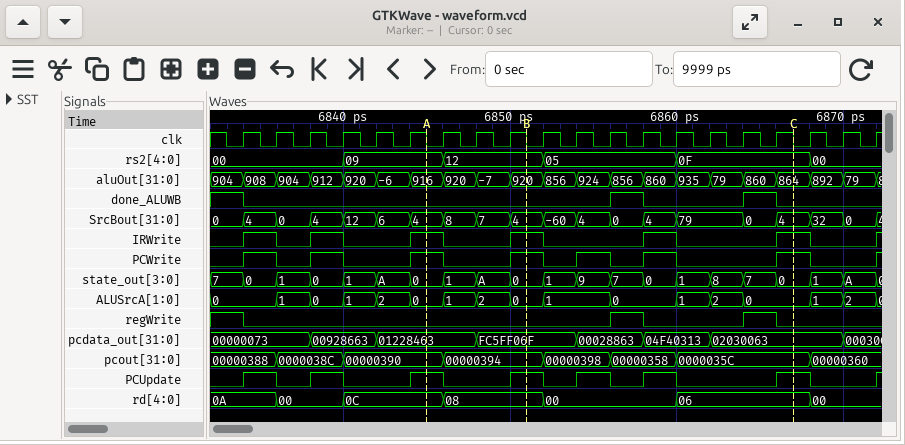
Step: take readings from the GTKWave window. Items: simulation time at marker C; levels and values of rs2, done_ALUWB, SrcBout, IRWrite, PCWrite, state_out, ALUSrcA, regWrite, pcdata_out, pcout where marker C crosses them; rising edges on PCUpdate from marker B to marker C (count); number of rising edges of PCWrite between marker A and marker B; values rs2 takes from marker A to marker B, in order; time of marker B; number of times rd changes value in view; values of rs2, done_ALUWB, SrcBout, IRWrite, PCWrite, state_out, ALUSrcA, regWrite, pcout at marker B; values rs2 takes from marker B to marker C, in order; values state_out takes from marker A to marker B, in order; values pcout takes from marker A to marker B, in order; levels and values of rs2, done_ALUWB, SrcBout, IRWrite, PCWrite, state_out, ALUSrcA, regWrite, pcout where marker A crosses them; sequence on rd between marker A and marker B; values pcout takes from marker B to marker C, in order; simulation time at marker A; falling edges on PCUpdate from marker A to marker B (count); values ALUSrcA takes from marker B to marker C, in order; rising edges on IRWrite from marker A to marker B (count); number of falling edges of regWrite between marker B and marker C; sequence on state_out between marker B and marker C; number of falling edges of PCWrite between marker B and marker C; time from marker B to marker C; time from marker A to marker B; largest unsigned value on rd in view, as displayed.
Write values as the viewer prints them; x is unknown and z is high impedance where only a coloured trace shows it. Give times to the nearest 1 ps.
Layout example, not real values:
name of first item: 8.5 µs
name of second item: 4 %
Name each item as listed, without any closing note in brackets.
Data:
simulation time at marker C: 6867 ps
levels and values of rs2, done_ALUWB, SrcBout, IRWrite, PCWrite, state_out, ALUSrcA, regWrite, pcdata_out, pcout where marker C crosses them: rs2=0F, done_ALUWB=0, SrcBout=4, IRWrite=1, PCWrite=1, state_out=0, ALUSrcA=0, regWrite=0, pcdata_out=02030063, pcout=0000035C
rising edges on PCUpdate from marker B to marker C: 3
number of rising edges of PCWrite between marker A and marker B: 1
values rs2 takes from marker A to marker B, in order: 09, 12
time of marker B: 6851 ps
number of times rd changes value in view: 6
values of rs2, done_ALUWB, SrcBout, IRWrite, PCWrite, state_out, ALUSrcA, regWrite, pcout at marker B: rs2=12, done_ALUWB=0, SrcBout=4, IRWrite=1, PCWrite=1, state_out=0, ALUSrcA=0, regWrite=0, pcout=00000394
values rs2 takes from marker B to marker C, in order: 12, 05, 0F
values state_out takes from marker A to marker B, in order: 0, 1, A, 0
values pcout takes from marker A to marker B, in order: 00000390, 00000394
levels and values of rs2, done_ALUWB, SrcBout, IRWrite, PCWrite, state_out, ALUSrcA, regWrite, pcout where marker A crosses them: rs2=09, done_ALUWB=0, SrcBout=4, IRWrite=1, PCWrite=1, state_out=0, ALUSrcA=0, regWrite=0, pcout=00000390
sequence on rd between marker A and marker B: 0C, 08
values pcout takes from marker B to marker C, in order: 00000394, 00000398, 00000358, 0000035C
simulation time at marker A: 6845 ps
falling edges on PCUpdate from marker A to marker B: 1
values ALUSrcA takes from marker B to marker C, in order: 0, 1, 0, 1, 2, 0
rising edges on IRWrite from marker A to marker B: 1
number of falling edges of regWrite between marker B and marker C: 2
sequence on state_out between marker B and marker C: 0, 1, 9, 7, 0, 1, 8, 7, 0
number of falling edges of PCWrite between marker B and marker C: 3
time from marker B to marker C: 16 ps
time from marker A to marker B: 6 ps
largest unsigned value on rd in view, as displayed: 0C
